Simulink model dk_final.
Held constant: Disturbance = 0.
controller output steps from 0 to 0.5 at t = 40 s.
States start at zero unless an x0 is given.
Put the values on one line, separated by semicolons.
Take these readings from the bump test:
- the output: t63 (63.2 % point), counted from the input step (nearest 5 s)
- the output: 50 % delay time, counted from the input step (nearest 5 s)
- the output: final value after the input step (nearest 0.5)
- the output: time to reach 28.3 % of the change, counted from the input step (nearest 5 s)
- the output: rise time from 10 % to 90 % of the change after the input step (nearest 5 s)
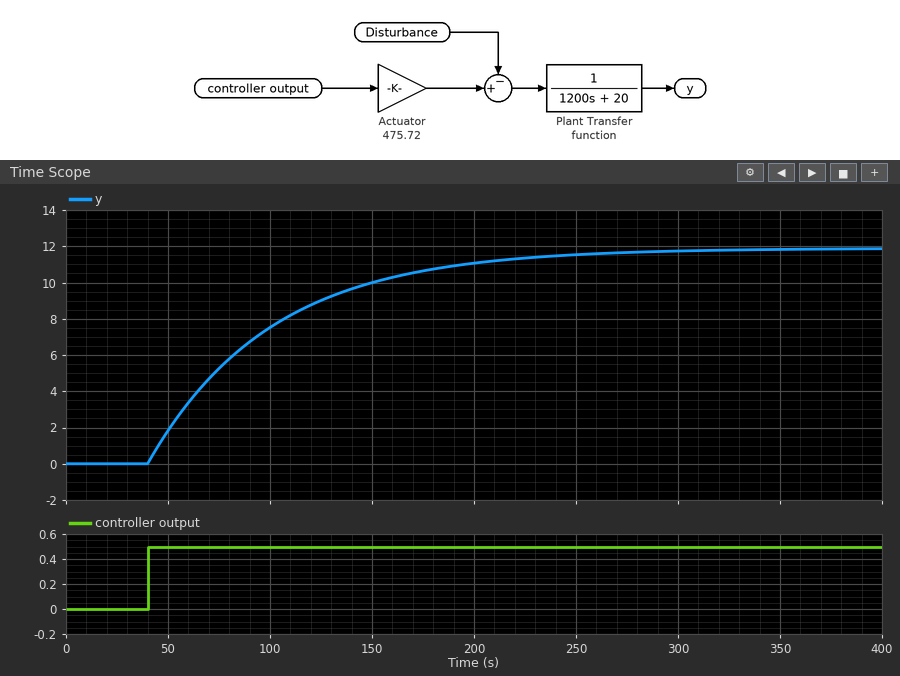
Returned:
60 s; 40 s; 12.0; 20 s; 130 s
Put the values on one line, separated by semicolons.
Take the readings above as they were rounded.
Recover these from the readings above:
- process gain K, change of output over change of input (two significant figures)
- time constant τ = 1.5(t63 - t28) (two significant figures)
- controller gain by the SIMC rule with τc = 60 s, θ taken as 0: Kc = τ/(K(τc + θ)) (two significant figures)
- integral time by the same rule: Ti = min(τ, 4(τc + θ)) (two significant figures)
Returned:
24; 60 s; 0.042; 60 s
